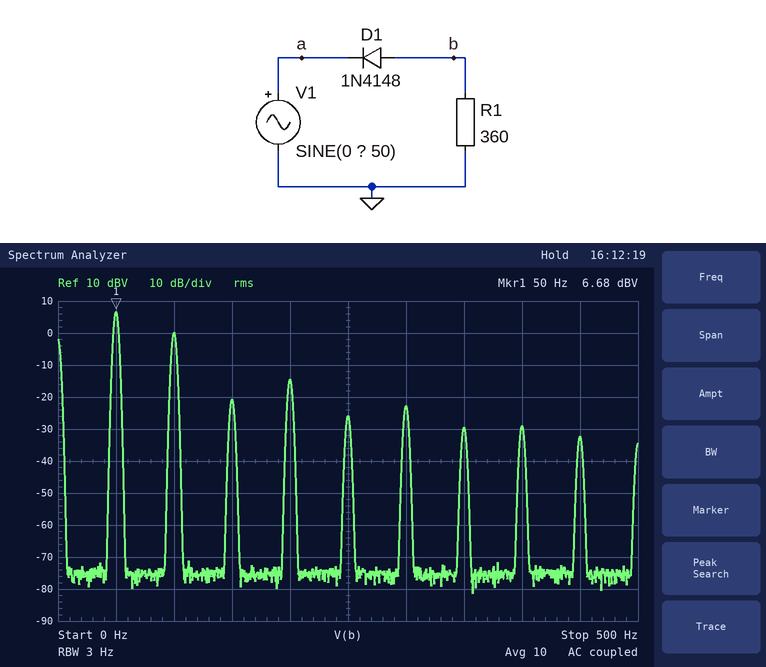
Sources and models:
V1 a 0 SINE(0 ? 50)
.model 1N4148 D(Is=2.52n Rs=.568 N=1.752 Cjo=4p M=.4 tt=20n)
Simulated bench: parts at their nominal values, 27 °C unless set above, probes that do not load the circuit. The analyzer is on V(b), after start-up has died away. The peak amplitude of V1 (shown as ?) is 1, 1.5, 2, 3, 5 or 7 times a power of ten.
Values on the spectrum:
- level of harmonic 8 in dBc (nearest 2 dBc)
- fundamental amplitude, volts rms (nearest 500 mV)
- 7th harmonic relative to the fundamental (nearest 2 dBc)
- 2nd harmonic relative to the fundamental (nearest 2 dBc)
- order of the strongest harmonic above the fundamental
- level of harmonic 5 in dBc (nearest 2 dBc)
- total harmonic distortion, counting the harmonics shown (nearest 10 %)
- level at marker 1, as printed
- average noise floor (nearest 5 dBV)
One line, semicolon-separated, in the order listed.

-36 dBc; 2.0 V; -36 dBc; -6 dBc; 2; -32 dBc; 50 %; 6.68 dBV; -75 dBV
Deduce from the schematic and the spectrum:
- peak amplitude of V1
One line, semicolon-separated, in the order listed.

7 V
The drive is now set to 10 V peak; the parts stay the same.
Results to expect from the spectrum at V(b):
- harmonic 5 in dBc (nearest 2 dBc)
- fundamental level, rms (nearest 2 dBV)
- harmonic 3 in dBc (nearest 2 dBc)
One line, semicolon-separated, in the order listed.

-36 dBc; 10 dBV; -30 dBc
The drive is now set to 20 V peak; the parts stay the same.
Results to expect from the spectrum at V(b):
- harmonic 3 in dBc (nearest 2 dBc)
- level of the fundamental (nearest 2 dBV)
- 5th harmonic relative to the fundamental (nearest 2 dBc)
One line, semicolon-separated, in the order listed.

-36 dBc; 16 dBV; -42 dBc
